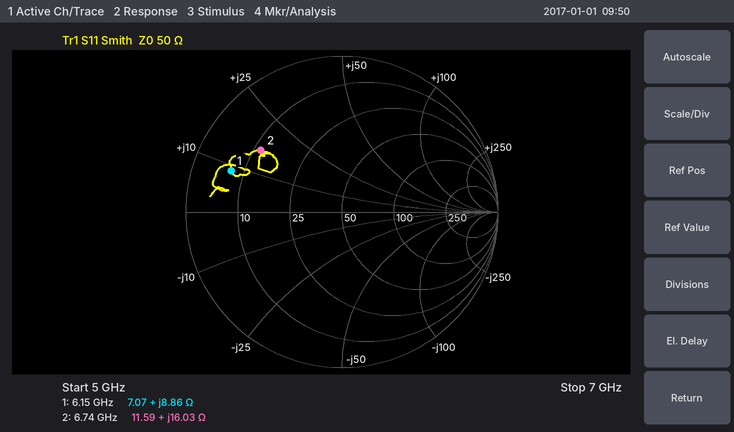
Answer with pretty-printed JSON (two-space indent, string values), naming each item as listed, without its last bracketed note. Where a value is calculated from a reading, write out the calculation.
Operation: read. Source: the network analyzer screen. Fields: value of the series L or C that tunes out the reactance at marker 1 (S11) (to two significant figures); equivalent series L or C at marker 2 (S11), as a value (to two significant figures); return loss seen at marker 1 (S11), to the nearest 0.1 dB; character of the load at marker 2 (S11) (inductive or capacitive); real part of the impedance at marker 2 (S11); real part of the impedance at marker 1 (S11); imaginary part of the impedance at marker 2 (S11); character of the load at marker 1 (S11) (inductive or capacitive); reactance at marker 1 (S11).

{
  "value of the series L or C that tunes out the reactance at marker 1 (S11)": "C = 1/(2π × 6.15 GHz × 8.86 Ω) ≈ 2.9 pF",
  "equivalent series L or C at marker 2 (S11), as a value": "L = 16.03 Ω/(2π × 6.74 GHz) ≈ 379 pH, so 380 pH to two significant figures",
  "return loss seen at marker 1 (S11), to the nearest 0.1 dB": "2.4 dB",
  "character of the load at marker 2 (S11)": "inductive",
  "real part of the impedance at marker 2": "11.59 Ω",
  "real part of the impedance at marker 1": "7.07 Ω",
  "imaginary part of the impedance at marker 2": "+16.03 Ω",
  "character of the load at marker 1 (S11)": "inductive",
  "reactance at marker 1": "+8.86 Ω"
}
